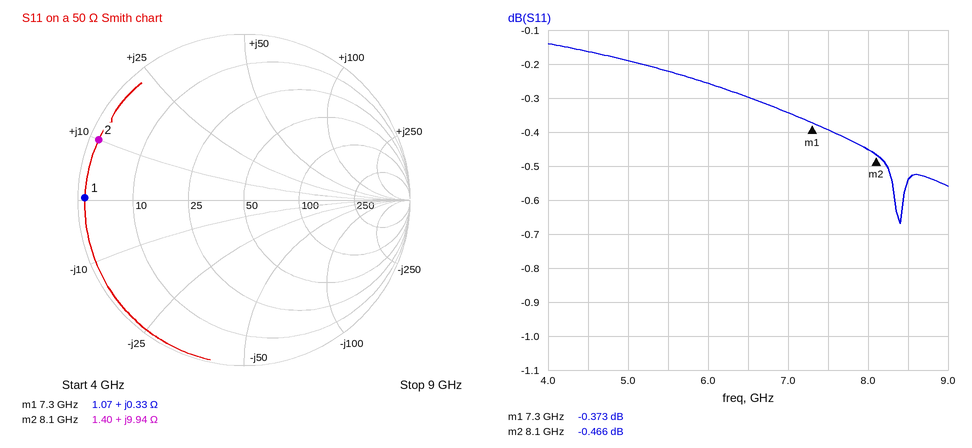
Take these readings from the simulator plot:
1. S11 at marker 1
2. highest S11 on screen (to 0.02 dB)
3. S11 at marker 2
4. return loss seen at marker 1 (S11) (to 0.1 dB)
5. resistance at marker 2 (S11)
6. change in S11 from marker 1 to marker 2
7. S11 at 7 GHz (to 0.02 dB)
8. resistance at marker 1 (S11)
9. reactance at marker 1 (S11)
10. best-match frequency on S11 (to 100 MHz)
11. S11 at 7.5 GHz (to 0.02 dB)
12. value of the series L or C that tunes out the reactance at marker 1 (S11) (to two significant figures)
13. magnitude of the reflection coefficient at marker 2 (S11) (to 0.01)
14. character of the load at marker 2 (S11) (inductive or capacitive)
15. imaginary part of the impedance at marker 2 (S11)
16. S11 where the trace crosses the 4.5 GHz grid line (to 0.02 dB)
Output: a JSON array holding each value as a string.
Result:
["-0.373 dB", "-0.14 dB", "-0.466 dB", "0.4 dB", "1.40 Ω", "-0.093 dB", "-0.34 dB", "1.07 Ω", "+0.33 Ω", "8.4 GHz", "-0.40 dB", "66 pF", "0.95", "inductive", "+9.94 Ω", "-0.16 dB"]
